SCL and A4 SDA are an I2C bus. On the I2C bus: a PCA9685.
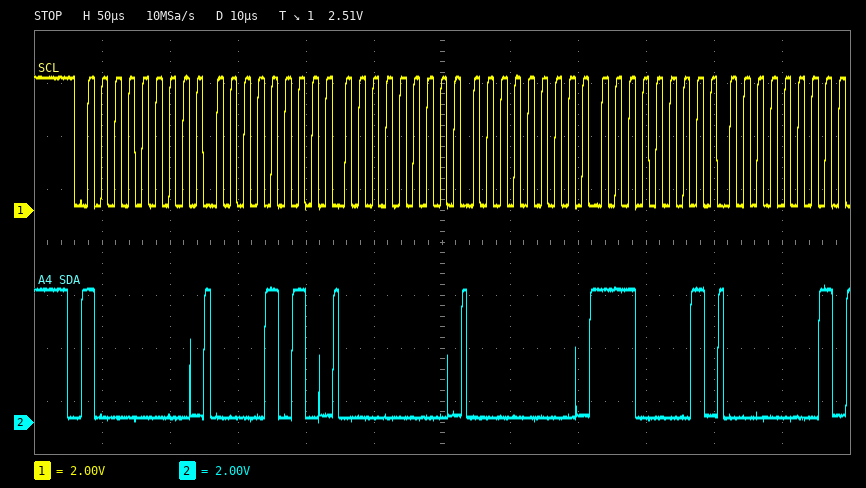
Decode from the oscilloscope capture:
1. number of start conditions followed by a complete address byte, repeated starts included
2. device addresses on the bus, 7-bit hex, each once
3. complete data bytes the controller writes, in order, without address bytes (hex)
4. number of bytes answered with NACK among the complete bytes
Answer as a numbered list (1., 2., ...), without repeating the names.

1. 1
2. 0x40
3. 0A 00 00 E1 01
4. 0
